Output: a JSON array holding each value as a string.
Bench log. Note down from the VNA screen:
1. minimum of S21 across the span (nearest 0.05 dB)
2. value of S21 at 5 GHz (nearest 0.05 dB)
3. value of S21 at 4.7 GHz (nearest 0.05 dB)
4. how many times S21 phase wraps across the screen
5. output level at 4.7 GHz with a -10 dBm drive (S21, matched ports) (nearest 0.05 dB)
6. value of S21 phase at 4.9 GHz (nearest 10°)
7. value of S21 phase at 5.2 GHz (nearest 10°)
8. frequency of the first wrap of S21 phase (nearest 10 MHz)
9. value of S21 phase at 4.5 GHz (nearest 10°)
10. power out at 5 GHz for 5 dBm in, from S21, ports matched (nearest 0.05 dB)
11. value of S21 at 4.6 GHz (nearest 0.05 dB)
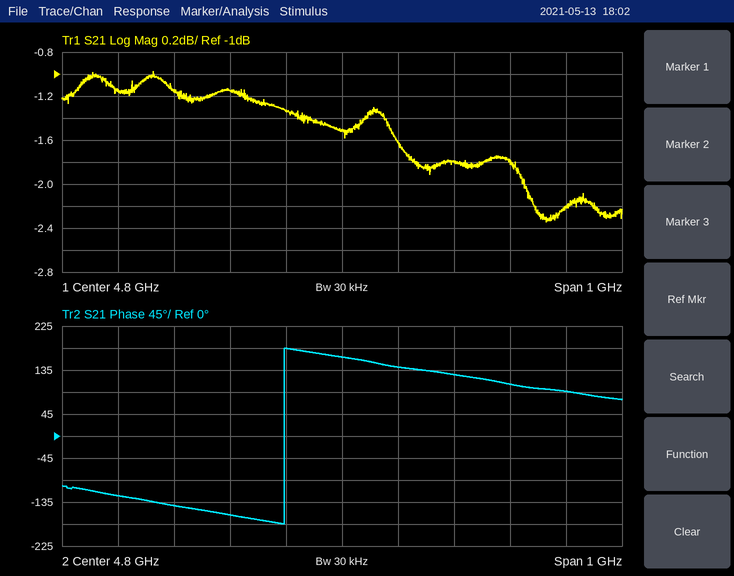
["-2.35 dB", "-1.80 dB", "-1.35 dB", "1", "-11.35 dBm", "140°", "90°", "4.70 GHz", "-140°", "3.20 dBm", "-1.15 dB"]
